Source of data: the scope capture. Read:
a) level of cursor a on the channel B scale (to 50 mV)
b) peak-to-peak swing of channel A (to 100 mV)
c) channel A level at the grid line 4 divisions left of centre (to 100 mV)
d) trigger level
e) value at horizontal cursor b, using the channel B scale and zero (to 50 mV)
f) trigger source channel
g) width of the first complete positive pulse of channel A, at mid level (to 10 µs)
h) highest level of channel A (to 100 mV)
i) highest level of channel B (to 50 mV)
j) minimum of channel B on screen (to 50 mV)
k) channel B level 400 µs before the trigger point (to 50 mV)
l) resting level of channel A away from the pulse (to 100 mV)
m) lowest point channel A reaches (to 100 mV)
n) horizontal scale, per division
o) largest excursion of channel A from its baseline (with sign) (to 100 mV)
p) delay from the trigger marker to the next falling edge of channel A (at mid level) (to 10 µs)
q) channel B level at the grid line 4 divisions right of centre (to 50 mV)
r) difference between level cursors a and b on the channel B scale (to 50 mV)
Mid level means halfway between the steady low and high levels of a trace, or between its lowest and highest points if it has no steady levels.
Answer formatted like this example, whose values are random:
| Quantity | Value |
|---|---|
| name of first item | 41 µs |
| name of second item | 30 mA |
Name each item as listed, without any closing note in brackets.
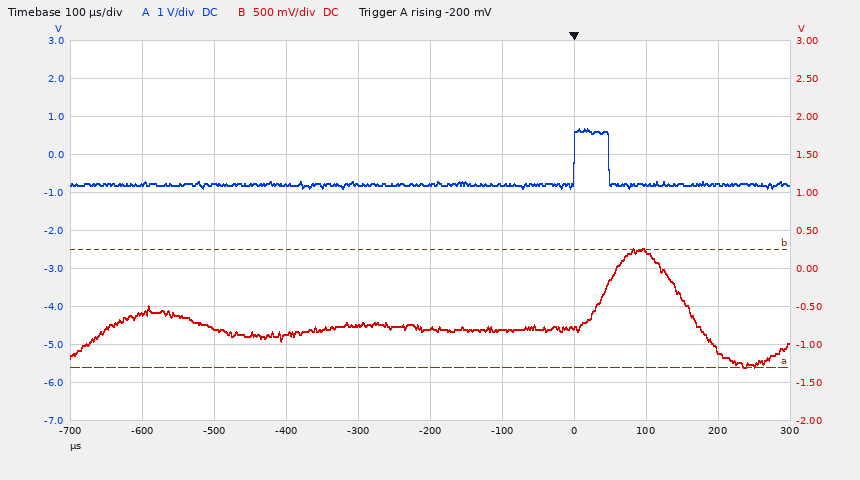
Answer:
| Quantity | Value |
|---|---|
| level of cursor a on the channel B scale | -1.30 V |
| peak-to-peak swing of channel A | 1.6 V |
| channel A level at the grid line 4 divisions left of centre | -800 mV |
| trigger level | -200 mV |
| value at horizontal cursor b, using the channel B scale and zero | 250 mV |
| trigger source channel | channel A |
| width of the first complete positive pulse of channel A, at mid level | 50 µs |
| highest level of channel A | 700 mV |
| highest level of channel B | 250 mV |
| minimum of channel B on screen | -1.30 V |
| channel B level 400 µs before the trigger point | -850 mV |
| resting level of channel A away from the pulse | -800 mV |
| lowest point channel A reaches | -900 mV |
| horizontal scale, per division | 100 µs |
| largest excursion of channel A from its baseline (with sign) | +1.5 V |
| delay from the trigger marker to the next falling edge of channel A (at mid level) | 50 µs |
| channel B level at the grid line 4 divisions right of centre | -1.05 V |
| difference between level cursors a and b on the channel B scale | 1.55 V |
